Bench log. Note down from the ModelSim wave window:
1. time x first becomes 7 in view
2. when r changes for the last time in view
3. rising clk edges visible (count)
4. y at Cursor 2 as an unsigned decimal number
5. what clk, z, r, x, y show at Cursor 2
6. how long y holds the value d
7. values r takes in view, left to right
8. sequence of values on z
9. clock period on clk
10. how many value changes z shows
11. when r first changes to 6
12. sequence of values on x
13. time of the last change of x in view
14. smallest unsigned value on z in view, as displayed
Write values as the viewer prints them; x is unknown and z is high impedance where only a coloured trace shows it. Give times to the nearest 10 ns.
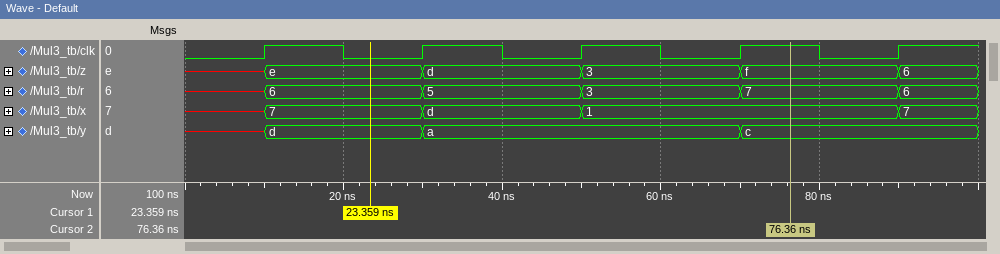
10 ns
90 ns
5
12
clk=1, z=f, r=7, x=1, y=c
20 ns
x, 6, 5, 3, 7, 6
x, e, d, 3, f, 6
20 ns
5
10 ns
x, 7, d, 1, 7
90 ns
3
